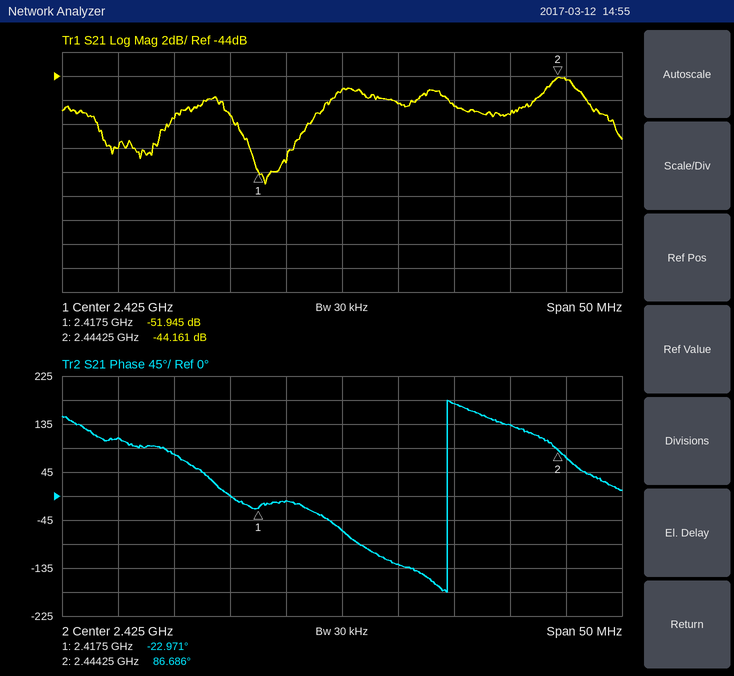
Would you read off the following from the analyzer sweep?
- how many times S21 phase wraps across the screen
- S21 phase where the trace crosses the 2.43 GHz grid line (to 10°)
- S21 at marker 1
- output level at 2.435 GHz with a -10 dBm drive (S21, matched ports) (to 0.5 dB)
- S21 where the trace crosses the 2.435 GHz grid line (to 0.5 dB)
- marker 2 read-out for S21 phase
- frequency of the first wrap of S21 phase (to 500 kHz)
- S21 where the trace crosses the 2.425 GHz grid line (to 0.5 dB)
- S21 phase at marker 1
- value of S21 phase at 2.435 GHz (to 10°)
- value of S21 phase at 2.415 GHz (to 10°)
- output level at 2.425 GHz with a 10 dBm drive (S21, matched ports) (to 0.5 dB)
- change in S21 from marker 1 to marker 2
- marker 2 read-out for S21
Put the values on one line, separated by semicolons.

1; -130°; -51.945 dB; -56.5 dBm; -46.5 dB; 86.686°; 2.4345 GHz; -45.0 dB; -22.971°; 170°; 0°; -35.0 dBm; 7.784 dB; -44.161 dB
